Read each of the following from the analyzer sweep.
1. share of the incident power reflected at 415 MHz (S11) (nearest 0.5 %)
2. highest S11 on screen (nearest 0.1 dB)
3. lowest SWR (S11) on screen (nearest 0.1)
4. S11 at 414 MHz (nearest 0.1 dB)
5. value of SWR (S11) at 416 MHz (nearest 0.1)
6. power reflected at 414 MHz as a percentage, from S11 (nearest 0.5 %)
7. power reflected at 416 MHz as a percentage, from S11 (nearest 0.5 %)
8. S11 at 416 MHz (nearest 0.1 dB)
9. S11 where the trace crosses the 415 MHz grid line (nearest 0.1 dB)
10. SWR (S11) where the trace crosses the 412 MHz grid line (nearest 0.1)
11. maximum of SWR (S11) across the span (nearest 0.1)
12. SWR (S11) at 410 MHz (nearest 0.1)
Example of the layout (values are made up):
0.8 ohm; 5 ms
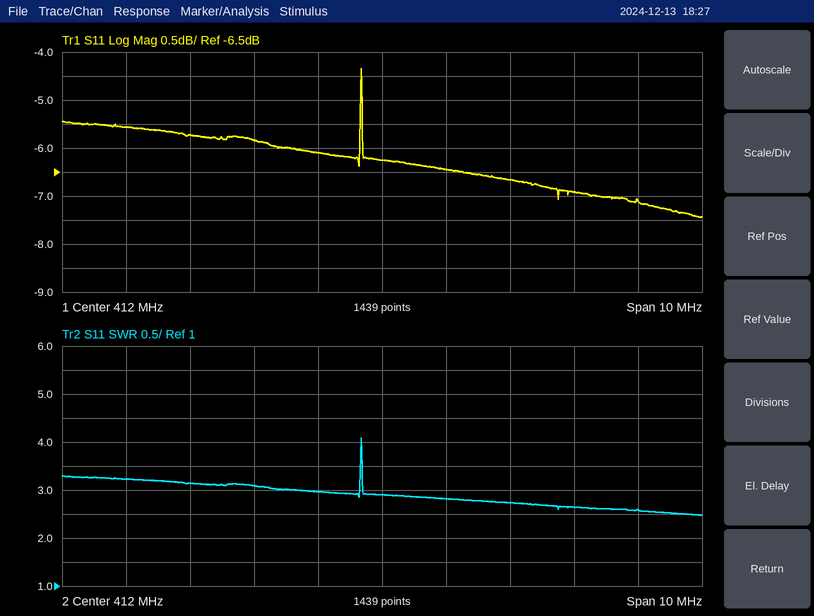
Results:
20.5 %; -4.3 dB; 2.5; -6.7 dB; 2.6; 21.5 %; 19.5 %; -7.1 dB; -6.9 dB; 2.9; 4.1; 3.1
